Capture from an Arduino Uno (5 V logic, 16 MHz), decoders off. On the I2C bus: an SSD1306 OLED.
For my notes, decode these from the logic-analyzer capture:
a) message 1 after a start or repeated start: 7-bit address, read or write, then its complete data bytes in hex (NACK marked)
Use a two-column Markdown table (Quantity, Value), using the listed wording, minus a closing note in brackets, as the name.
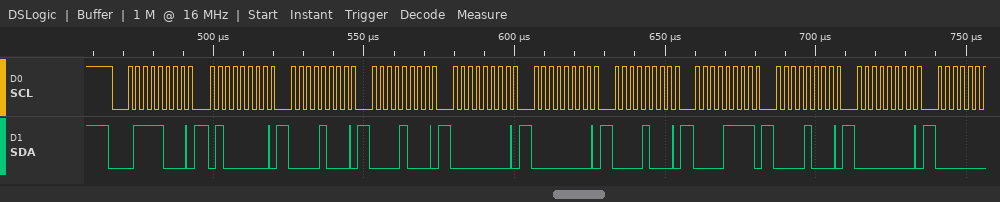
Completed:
| Quantity | Value |
|---|---|
| message 1 after a start or repeated start: 7-bit address, read or write, then its complete data bytes in hex | 0x3C write: 40 08 08 00 00 08 0F 08 00 |
